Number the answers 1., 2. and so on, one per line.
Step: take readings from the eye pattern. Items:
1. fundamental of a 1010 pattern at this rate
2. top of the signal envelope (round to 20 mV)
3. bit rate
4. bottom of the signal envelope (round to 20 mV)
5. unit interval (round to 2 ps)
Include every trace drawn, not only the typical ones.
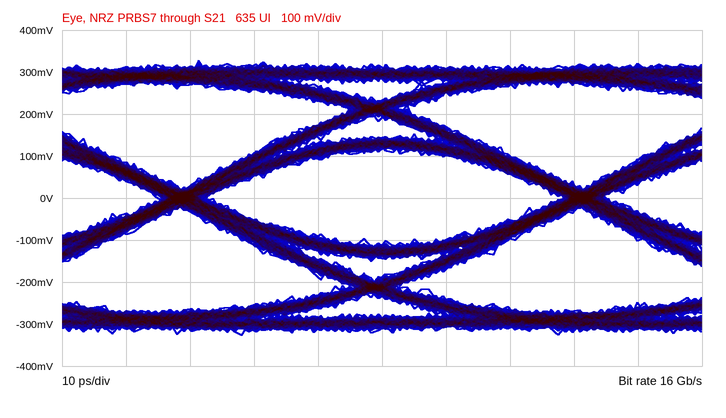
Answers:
1. 8 GHz
2. 320 mV
3. 16 Gb/s
4. -320 mV
5. 62 ps
